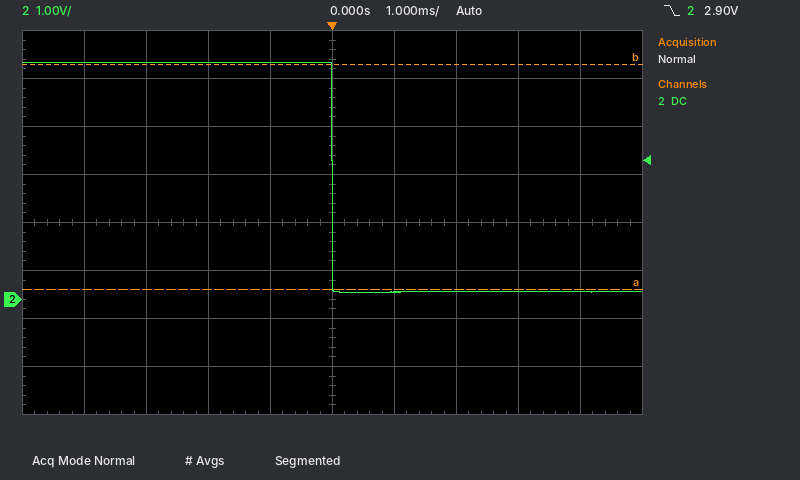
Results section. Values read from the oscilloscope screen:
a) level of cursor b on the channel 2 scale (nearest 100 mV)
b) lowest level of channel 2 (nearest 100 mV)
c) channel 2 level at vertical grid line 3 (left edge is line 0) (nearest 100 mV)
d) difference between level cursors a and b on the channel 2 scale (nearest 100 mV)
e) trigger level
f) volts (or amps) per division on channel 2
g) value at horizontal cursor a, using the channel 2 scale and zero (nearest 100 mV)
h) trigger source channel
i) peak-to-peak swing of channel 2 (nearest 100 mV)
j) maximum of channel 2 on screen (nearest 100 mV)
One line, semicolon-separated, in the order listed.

4.9 V; 100 mV; 4.9 V; 4.7 V; 2.90 V; 1 V; 200 mV; channel 2; 4.8 V; 4.9 V
